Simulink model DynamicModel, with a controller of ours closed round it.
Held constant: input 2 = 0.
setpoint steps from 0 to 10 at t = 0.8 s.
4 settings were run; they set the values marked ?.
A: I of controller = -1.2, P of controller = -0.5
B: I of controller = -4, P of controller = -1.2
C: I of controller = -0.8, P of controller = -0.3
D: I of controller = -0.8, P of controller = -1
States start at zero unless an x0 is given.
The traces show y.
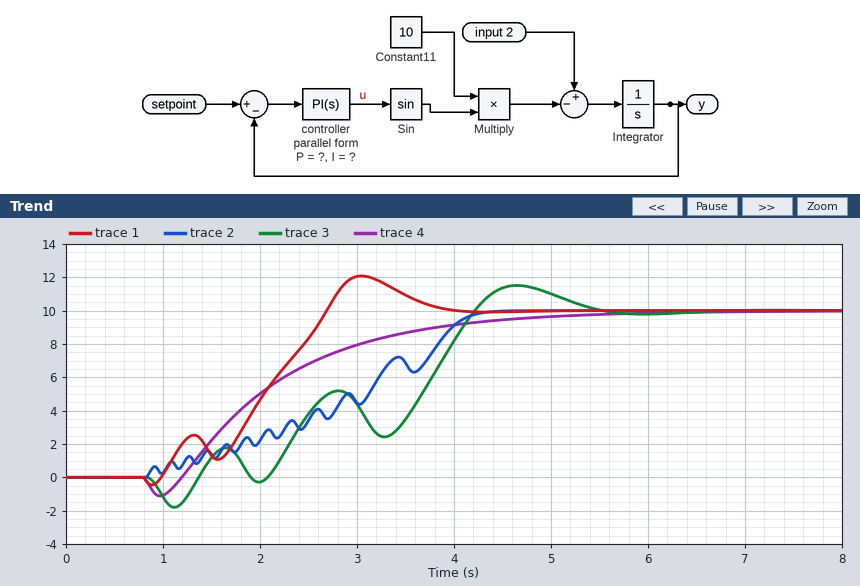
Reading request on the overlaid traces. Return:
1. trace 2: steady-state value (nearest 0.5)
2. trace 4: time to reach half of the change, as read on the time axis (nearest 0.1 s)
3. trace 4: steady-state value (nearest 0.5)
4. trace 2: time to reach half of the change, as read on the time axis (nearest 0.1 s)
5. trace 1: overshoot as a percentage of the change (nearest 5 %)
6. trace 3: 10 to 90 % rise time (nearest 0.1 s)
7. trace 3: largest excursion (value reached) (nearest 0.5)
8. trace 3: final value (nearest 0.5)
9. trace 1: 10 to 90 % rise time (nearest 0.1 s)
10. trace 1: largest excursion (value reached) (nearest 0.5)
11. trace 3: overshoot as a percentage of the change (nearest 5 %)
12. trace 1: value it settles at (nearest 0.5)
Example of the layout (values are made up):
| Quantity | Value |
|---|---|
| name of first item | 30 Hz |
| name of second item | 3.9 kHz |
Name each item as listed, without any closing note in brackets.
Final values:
| Quantity | Value |
|---|---|
| trace 2: steady-state value | 10.0 |
| trace 4: time to reach half of the change, as read on the time axis | 2.0 s |
| trace 4: steady-state value | 10.0 |
| trace 2: time to reach half of the change, as read on the time axis | 2.9 s |
| trace 1: overshoot as a percentage of the change | 20 % |
| trace 3: 10 to 90 % rise time | 2.6 s |
| trace 3: largest excursion (value reached) | 11.5 |
| trace 3: final value | 10.0 |
| trace 1: 10 to 90 % rise time | 1.5 s |
| trace 1: largest excursion (value reached) | 12.0 |
| trace 3: overshoot as a percentage of the change | 15 % |
| trace 1: value it settles at | 10.0 |
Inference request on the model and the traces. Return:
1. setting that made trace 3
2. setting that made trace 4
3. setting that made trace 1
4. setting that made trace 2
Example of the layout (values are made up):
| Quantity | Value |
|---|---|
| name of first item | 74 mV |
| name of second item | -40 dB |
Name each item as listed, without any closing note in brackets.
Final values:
| Quantity | Value |
|---|---|
| setting that made trace 3 | C |
| setting that made trace 4 | D |
| setting that made trace 1 | A |
| setting that made trace 2 | B |
